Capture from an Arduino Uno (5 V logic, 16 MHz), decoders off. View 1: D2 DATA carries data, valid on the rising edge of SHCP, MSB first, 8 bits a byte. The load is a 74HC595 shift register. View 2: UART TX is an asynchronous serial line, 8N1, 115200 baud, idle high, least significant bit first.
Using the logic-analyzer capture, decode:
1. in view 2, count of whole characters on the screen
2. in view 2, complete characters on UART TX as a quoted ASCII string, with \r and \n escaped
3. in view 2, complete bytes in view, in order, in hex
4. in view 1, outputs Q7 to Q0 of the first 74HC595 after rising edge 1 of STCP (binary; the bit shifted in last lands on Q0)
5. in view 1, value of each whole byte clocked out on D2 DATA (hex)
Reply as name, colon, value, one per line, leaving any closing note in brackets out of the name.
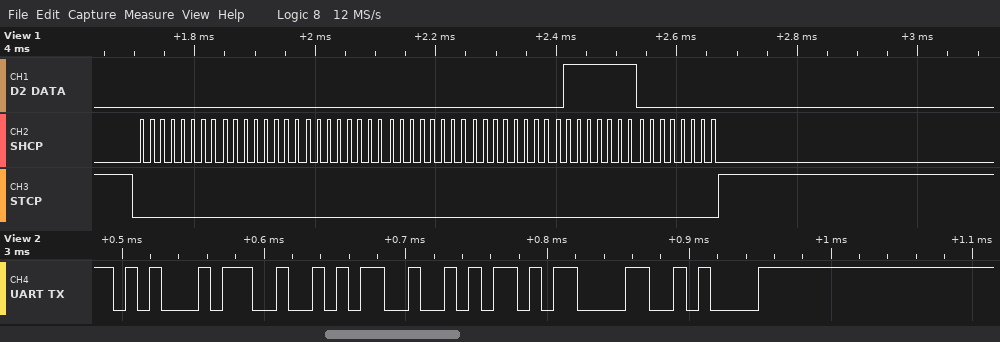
in view 2, count of whole characters on the screen: 5
in view 2, complete characters on UART TX as a quoted ASCII string, with \r and \n escaped: "ERR\r\n"
in view 2, complete bytes in view, in order, in hex: 0x45 0x52 0x52 0x0D 0x0A
in view 1, outputs Q7 to Q0 of the first 74HC595 after rising edge 1 of STCP: 00000000
in view 1, value of each whole byte clocked out on D2 DATA: 00 00 00 00 00 7F 00
